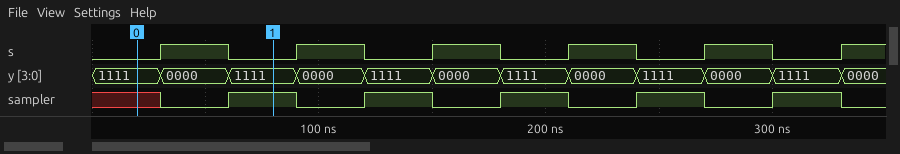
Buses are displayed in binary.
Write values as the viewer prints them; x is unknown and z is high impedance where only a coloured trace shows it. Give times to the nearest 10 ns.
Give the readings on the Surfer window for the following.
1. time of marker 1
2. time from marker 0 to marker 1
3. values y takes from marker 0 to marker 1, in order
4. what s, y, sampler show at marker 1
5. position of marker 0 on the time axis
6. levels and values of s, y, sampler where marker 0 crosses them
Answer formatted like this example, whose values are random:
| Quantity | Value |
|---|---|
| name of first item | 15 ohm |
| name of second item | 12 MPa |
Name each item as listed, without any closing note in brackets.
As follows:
| Quantity | Value |
|---|---|
| time of marker 1 | 80 ns |
| time from marker 0 to marker 1 | 60 ns |
| values y takes from marker 0 to marker 1, in order | 1111, 0000, 1111 |
| what s, y, sampler show at marker 1 | s=0, y=1111, sampler=1 |
| position of marker 0 on the time axis | 20 ns |
| levels and values of s, y, sampler where marker 0 crosses them | s=0, y=1111, sampler=x |
